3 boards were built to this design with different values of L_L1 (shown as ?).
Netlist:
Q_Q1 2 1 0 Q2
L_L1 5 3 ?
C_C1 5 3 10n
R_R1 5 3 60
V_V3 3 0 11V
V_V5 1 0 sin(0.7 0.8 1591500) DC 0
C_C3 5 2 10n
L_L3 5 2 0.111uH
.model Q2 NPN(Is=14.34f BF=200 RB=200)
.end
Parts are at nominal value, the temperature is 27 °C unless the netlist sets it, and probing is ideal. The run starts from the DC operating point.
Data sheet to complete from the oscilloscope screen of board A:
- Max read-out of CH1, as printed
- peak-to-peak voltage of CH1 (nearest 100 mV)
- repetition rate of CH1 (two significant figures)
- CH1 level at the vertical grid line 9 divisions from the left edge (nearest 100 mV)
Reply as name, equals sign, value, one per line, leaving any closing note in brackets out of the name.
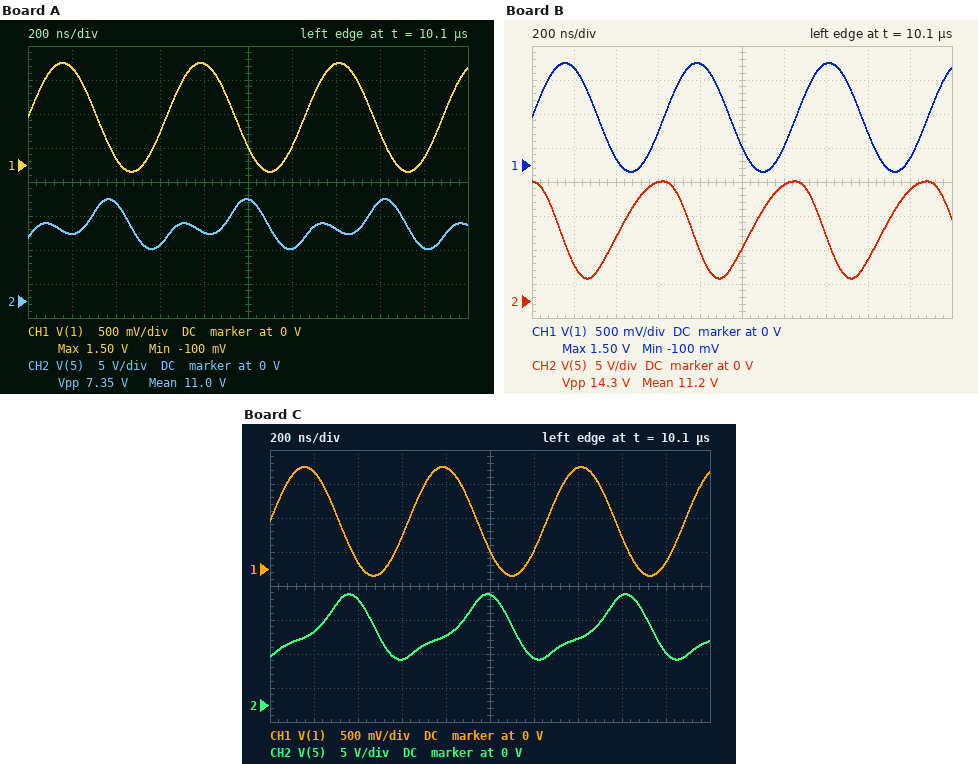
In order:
Max read-out of CH1, as printed = 1.50 V
peak-to-peak voltage of CH1 = 1.6 V
repetition rate of CH1 = 1.6 MHz
CH1 level at the vertical grid line 9 divisions from the left edge = 100 mV
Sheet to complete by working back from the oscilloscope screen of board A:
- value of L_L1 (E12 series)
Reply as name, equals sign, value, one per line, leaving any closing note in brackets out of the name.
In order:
value of L_L1 = 390 nH
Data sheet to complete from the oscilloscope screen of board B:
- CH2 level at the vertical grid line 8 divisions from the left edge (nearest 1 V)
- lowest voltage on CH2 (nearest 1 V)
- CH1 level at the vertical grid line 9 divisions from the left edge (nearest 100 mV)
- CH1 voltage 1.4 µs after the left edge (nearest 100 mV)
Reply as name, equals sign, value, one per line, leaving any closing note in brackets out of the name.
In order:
CH2 level at the vertical grid line 8 divisions from the left edge = 6 V
lowest voltage on CH2 = 3 V
CH1 level at the vertical grid line 9 divisions from the left edge = 100 mV
CH1 voltage 1.4 µs after the left edge = 1.5 V
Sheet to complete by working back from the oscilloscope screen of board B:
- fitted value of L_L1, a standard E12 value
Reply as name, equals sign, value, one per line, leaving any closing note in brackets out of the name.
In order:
fitted value of L_L1, a standard E12 value = 1.8 µH
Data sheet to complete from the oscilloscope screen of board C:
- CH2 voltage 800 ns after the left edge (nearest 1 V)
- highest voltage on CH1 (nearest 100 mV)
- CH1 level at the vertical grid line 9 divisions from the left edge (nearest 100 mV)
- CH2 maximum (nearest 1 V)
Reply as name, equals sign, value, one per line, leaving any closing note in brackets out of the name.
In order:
CH2 voltage 800 ns after the left edge = 10 V
highest voltage on CH1 = 1.5 V
CH1 level at the vertical grid line 9 divisions from the left edge = 100 mV
CH2 maximum = 16 V
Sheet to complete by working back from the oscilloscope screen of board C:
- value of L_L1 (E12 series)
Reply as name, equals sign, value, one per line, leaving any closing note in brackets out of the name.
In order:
value of L_L1 = 560 nH
